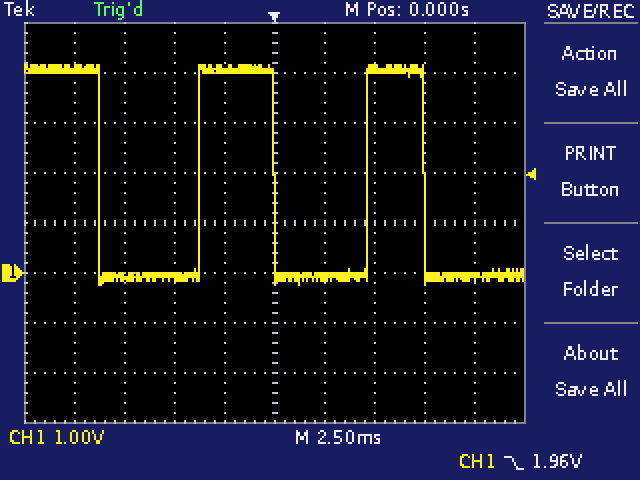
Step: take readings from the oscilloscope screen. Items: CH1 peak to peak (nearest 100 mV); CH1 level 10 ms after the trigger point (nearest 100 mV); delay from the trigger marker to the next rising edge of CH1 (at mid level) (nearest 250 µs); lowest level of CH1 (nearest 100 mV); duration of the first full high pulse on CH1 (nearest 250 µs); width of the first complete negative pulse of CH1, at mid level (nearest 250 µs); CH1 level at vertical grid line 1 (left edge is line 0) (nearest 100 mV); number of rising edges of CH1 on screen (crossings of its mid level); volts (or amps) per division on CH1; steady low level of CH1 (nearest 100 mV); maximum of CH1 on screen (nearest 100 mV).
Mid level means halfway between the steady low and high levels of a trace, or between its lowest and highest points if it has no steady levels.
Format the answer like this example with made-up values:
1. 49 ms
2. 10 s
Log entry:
1. 4.4 V
2. -100 mV
3. 4.75 ms
4. -200 mV
5. 3.75 ms
6. 5.00 ms
7. 4.1 V
8. 2
9. 1 V
10. -100 mV
11. 4.2 V
